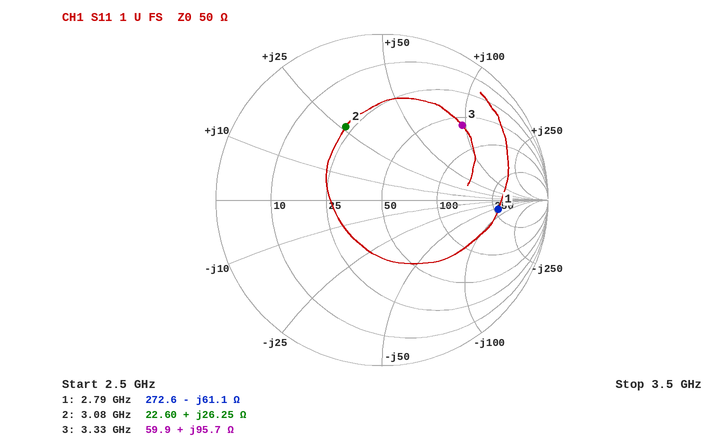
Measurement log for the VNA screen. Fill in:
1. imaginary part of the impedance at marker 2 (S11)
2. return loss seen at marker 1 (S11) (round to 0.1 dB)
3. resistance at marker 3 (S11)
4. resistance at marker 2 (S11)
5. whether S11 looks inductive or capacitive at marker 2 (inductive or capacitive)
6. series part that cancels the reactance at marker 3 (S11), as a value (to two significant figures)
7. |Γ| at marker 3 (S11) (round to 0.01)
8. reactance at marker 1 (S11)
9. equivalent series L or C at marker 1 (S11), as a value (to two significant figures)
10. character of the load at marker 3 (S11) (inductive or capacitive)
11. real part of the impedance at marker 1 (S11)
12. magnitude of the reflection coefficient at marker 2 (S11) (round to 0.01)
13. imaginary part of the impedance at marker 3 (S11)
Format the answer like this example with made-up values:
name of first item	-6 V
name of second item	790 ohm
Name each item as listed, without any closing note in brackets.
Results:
imaginary part of the impedance at marker 2	+26.25 Ω
return loss seen at marker 1 (S11)	3.1 dB
resistance at marker 3	59.9 Ω
resistance at marker 2	22.60 Ω
whether S11 looks inductive or capacitive at marker 2	inductive
series part that cancels the reactance at marker 3 (S11), as a value	500 fF
|Γ| at marker 3 (S11)	0.66
reactance at marker 1	-61.1 Ω
equivalent series L or C at marker 1 (S11), as a value	930 fF
character of the load at marker 3 (S11)	inductive
real part of the impedance at marker 1	272.6 Ω
magnitude of the reflection coefficient at marker 2 (S11)	0.49
imaginary part of the impedance at marker 3	+95.7 Ω
